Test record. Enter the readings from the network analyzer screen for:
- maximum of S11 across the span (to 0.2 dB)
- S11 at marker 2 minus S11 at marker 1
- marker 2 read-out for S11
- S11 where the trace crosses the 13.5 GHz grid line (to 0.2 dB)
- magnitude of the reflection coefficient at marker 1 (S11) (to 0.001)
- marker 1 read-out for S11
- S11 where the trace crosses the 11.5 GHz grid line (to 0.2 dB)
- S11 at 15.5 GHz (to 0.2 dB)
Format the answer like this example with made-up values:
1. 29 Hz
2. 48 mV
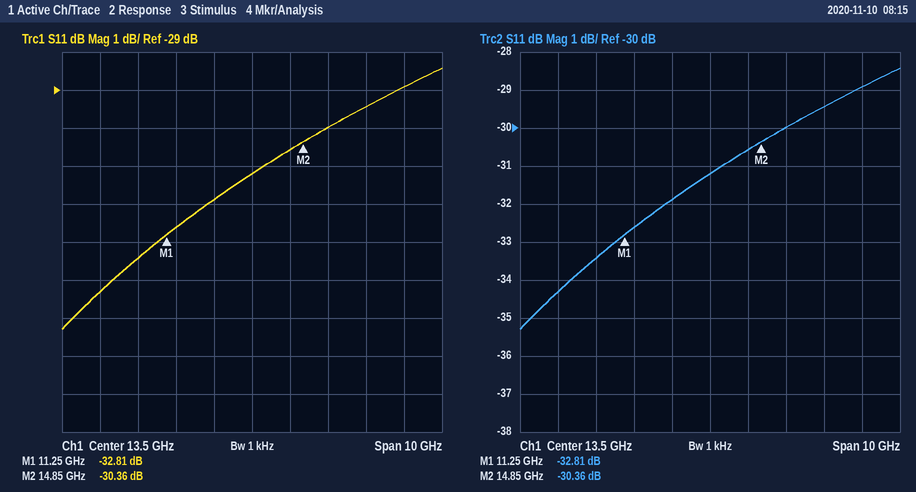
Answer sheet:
1. -28.4 dB
2. 2.45 dB
3. -30.36 dB
4. -31.2 dB
5. 0.023
6. -32.81 dB
7. -32.6 dB
8. -30.0 dB
